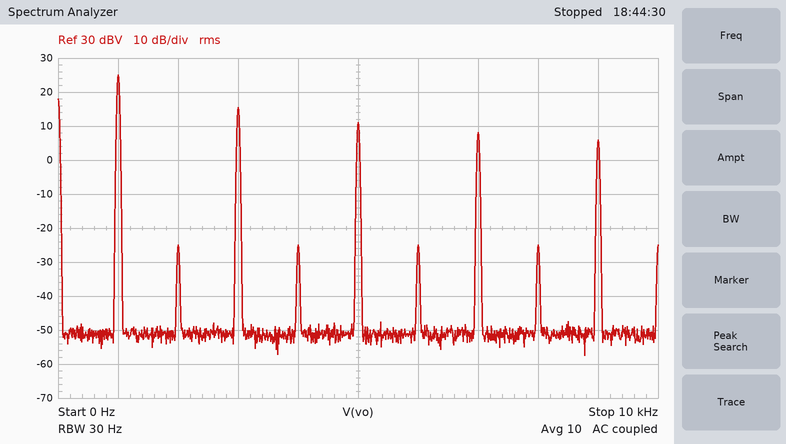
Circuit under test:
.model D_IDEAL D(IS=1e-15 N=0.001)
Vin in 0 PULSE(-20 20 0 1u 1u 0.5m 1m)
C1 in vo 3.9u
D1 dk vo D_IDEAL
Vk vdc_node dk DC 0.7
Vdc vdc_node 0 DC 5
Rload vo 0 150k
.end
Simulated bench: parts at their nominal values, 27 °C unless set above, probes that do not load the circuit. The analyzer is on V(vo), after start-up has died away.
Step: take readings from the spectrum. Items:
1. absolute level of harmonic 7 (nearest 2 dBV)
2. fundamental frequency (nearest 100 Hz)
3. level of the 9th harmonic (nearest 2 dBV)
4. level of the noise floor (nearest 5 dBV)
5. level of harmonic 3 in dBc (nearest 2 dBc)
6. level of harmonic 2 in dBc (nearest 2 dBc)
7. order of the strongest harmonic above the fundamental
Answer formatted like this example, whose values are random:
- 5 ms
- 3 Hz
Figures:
- 8 dBV
- 1.0 kHz
- 6 dBV
- -50 dBV
- -10 dBc
- -50 dBc
- 3
